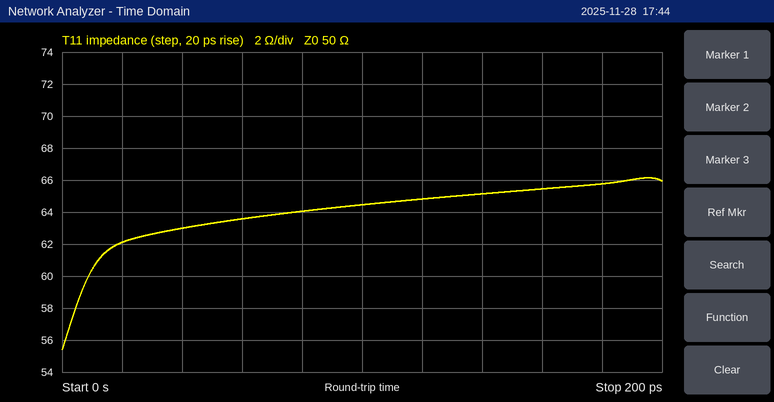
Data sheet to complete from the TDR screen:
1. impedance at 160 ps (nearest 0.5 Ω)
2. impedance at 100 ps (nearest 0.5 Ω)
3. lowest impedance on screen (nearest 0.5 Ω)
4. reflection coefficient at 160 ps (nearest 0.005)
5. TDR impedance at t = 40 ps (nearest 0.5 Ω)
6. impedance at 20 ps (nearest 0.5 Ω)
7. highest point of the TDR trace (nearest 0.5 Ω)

65.5 Ω
64.5 Ω
55.5 Ω
+0.135
63.0 Ω
62.0 Ω
66.0 Ω
